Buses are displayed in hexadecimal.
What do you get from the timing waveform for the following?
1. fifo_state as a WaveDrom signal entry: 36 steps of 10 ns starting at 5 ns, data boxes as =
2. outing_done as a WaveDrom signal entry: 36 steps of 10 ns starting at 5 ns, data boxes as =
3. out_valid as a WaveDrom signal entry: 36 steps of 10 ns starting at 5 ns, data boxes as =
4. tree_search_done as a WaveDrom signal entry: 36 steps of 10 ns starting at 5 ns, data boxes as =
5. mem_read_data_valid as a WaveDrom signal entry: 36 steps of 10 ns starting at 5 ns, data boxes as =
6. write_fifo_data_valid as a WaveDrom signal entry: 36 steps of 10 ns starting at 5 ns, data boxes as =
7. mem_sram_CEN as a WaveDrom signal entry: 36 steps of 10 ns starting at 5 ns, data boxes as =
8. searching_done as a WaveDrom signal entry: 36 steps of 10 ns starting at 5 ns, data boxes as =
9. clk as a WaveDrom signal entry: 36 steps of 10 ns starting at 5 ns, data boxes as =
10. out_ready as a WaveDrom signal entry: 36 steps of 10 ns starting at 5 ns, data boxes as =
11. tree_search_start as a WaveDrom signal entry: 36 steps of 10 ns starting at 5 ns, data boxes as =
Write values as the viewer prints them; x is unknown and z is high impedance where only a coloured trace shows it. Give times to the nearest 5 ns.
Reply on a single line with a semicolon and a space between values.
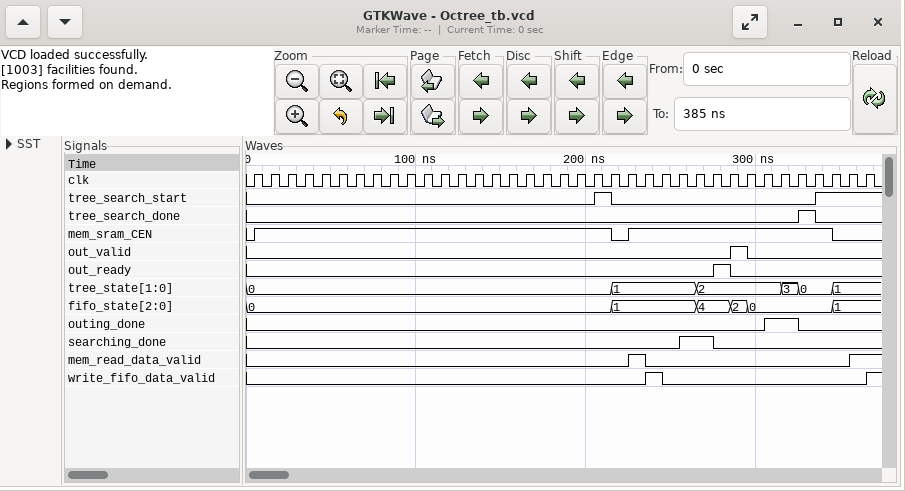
{name: 'fifo_state', wave: '=....................=....=.==....=.', data: '0 1 4 2 0 1'}; {name: 'outing_done', wave: '0.............................1.0...'}; {name: 'out_valid', wave: '0...........................10......'}; {name: 'tree_search_done', wave: '0...............................10..'}; {name: 'mem_read_data_valid', wave: '0.....................10...........1'}; {name: 'write_fifo_data_valid', wave: '0......................10...........'}; {name: 'mem_sram_CEN', wave: '1....................01...........0.'}; {name: 'searching_done', wave: '0........................1.0........'}; {name: 'clk', wave: 'p...................................'}; {name: 'out_ready', wave: '0..........................10.......'}; {name: 'tree_search_start', wave: '0...................10...........1..'}
